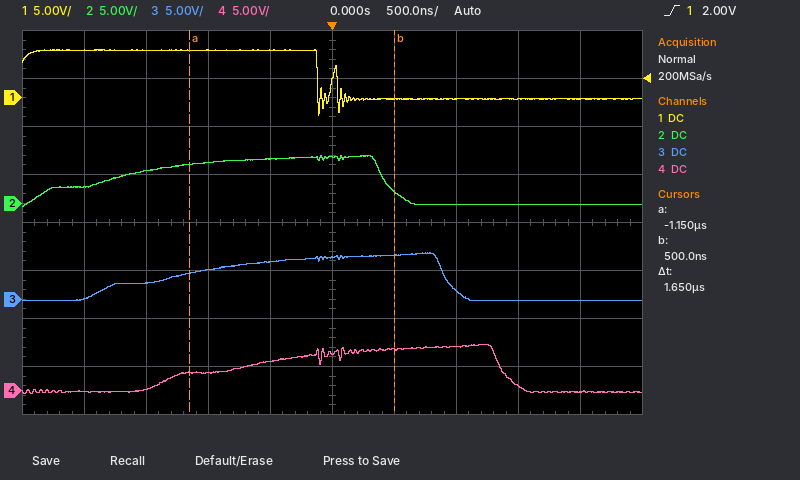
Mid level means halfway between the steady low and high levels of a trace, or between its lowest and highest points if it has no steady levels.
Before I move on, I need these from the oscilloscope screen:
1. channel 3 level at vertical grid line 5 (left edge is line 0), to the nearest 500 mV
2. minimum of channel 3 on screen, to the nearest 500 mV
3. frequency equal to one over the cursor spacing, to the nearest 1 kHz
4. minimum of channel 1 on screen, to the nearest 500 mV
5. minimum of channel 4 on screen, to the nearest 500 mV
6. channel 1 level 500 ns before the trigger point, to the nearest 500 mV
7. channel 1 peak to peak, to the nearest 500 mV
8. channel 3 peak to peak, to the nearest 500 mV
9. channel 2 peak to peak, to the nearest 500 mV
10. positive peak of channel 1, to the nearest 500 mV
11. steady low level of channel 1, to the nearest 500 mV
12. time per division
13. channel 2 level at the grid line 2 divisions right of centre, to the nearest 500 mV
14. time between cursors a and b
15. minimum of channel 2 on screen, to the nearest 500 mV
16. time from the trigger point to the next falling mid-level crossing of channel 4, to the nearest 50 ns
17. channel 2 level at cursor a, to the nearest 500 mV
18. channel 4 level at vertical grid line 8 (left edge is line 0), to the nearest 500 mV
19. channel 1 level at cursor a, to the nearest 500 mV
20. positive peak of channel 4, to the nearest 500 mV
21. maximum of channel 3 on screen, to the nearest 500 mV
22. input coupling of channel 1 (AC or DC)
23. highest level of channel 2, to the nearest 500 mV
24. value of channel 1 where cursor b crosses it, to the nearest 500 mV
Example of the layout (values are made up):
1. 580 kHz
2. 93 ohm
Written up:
1. 4.5 V
2. 0.0 V
3. 606 kHz
4. -2.0 V
5. -500 mV
6. 5.0 V
7. 7.0 V
8. 5.0 V
9. 5.5 V
10. 5.0 V
11. 0.0 V
12. 500 ns
13. 0.0 V
14. 1.65 µs
15. -500 mV
16. 1.35 µs
17. 4.0 V
18. 500 mV
19. 5.0 V
20. 5.0 V
21. 5.0 V
22. DC
23. 5.0 V
24. 0.0 V
